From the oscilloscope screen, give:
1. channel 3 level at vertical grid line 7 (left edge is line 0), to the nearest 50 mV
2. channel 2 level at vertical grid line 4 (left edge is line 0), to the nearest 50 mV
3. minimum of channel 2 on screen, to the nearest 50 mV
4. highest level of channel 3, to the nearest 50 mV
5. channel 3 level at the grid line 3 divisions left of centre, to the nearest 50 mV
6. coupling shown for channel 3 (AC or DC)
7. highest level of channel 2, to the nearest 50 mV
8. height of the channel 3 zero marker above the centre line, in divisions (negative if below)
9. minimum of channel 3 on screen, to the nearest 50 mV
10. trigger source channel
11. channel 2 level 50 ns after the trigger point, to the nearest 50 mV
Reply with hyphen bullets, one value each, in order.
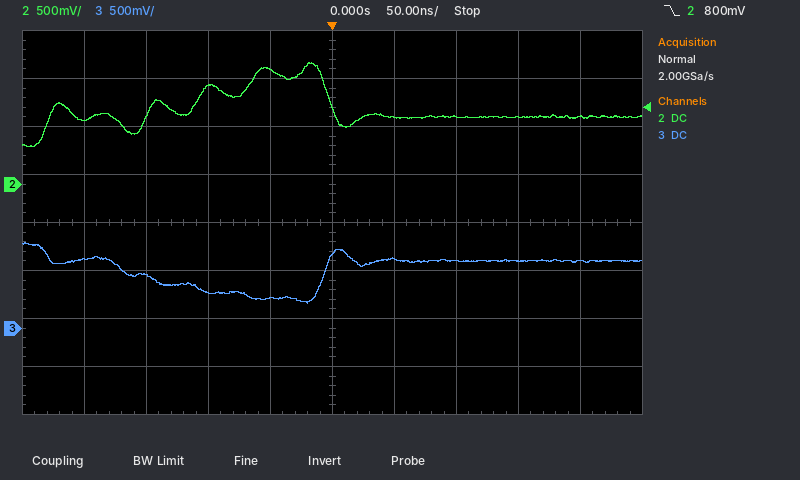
- 700 mV
- 1.20 V
- 400 mV
- 900 mV
- 550 mV
- DC
- 1.25 V
- -2.2 div
- 250 mV
- channel 2
- 700 mV
